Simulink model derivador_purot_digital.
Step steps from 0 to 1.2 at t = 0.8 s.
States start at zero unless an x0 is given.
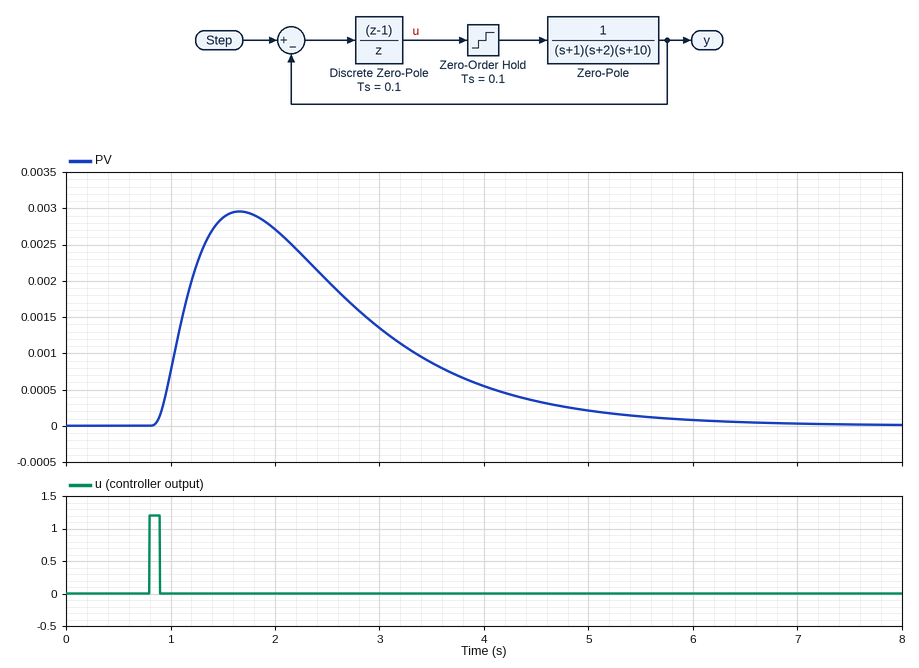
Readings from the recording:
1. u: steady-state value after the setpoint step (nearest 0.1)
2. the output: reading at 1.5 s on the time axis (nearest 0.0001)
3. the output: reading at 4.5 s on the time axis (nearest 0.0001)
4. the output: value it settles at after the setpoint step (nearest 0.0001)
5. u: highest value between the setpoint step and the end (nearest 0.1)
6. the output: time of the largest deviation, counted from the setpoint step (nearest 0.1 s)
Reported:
0.0
0.0029
0.0003
0.0000
1.2
0.9 s
